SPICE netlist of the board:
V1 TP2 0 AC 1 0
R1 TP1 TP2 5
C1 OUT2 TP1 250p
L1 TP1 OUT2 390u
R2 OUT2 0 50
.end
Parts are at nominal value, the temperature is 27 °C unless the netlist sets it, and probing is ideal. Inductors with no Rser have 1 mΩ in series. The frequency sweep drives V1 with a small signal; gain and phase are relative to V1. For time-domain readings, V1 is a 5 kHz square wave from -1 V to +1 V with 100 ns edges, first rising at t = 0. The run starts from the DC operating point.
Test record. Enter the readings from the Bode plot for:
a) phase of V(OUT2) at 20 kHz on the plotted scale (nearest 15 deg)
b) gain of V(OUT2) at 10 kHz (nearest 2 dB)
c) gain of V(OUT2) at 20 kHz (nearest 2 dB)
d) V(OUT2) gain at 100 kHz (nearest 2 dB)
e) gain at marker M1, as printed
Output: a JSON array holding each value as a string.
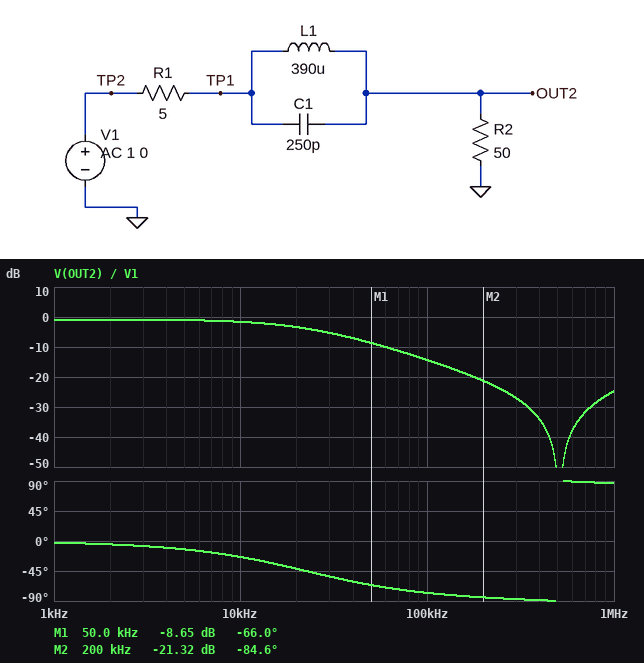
["-45 deg", "-2 dB", "-4 dB", "-14 dB", "-8.65 dB"]
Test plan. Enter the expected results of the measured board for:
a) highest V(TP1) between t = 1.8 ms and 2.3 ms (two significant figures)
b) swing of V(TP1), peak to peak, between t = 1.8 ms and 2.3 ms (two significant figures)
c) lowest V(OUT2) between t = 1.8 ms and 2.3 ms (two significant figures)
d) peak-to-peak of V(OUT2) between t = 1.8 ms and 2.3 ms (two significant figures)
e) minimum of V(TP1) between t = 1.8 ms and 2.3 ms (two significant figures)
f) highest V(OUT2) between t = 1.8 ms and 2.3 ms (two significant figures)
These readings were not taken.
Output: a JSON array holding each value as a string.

["1.1 V", "2.2 V", "-910 mV", "1.8 V", "-1.1 V", "910 mV"]
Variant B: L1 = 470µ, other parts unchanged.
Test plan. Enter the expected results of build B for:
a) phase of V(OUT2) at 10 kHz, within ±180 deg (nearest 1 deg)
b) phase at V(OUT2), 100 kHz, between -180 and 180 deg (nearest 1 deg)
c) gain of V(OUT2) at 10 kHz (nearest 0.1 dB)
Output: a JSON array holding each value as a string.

["-28 deg", "-80 deg", "-1.9 dB"]
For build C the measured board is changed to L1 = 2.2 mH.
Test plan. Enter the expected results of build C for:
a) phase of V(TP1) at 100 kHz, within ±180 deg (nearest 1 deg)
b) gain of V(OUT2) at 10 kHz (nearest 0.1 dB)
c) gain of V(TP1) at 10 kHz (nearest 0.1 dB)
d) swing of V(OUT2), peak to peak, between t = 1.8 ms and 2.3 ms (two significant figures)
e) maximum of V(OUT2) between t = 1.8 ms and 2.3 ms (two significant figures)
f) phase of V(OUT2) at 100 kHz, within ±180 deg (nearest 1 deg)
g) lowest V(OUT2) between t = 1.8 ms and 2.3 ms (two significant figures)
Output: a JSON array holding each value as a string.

["0 deg", "-9.5 dB", "-0.1 dB", "1.5 V", "770 mV", "-88 deg", "-770 mV"]
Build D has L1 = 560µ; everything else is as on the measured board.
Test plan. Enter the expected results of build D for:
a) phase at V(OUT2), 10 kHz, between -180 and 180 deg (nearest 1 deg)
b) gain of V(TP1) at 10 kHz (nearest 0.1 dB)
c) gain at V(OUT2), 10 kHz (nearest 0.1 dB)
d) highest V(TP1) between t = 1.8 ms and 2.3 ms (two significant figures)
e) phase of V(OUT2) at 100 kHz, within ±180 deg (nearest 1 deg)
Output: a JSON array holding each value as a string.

["-33 deg", "-0.6 dB", "-2.3 dB", "1.1 V", "-82 deg"]
